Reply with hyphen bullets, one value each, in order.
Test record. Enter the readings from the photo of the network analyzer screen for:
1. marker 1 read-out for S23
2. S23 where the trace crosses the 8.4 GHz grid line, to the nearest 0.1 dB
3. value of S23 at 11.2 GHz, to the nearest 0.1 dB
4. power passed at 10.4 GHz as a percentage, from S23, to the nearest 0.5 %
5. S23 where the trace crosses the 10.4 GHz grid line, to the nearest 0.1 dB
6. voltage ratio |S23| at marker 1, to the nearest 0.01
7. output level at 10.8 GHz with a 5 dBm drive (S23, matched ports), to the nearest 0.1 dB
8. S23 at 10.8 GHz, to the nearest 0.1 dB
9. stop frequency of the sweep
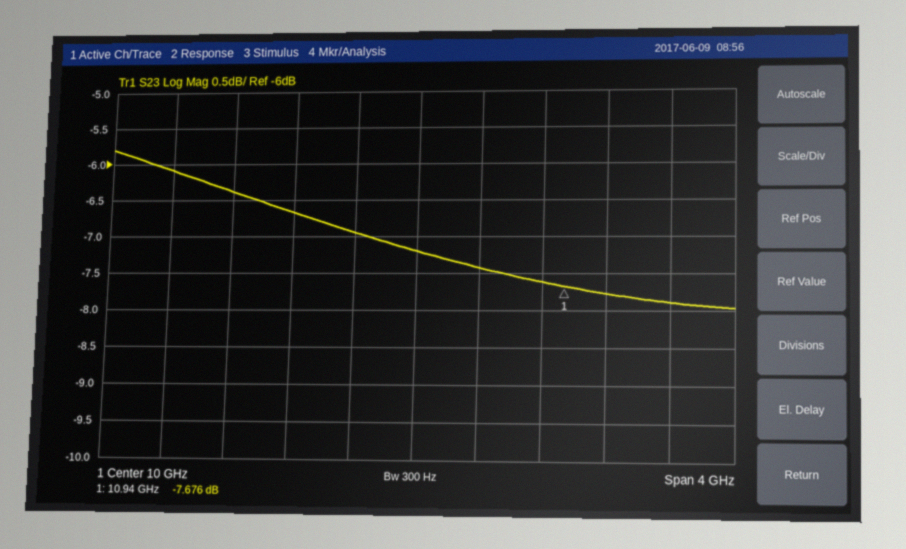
- -7.676 dB
- -6.1 dB
- -7.8 dB
- 18.0 %
- -7.4 dB
- 0.41
- -2.6 dBm
- -7.6 dB
- 12 GHz
